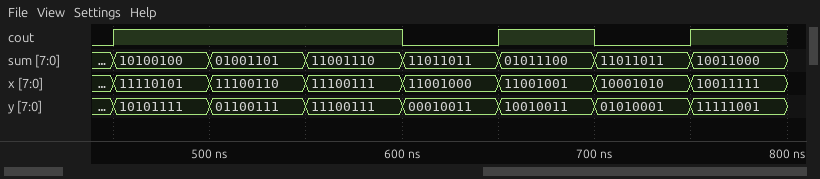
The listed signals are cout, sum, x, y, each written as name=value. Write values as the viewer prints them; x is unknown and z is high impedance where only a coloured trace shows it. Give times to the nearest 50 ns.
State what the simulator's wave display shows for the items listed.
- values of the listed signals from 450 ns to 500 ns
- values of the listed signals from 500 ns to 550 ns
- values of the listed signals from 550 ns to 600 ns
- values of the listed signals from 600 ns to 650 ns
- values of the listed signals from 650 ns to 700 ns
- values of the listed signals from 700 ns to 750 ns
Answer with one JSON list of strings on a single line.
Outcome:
["cout=1, sum=10100100, x=11110101, y=10101111", "cout=1, sum=01001101, x=11100110, y=01100111", "cout=1, sum=11001110, x=11100111, y=11100111", "cout=0, sum=11011011, x=11001000, y=00010011", "cout=1, sum=01011100, x=11001001, y=10010011", "cout=0, sum=11011011, x=10001010, y=01010001"]
